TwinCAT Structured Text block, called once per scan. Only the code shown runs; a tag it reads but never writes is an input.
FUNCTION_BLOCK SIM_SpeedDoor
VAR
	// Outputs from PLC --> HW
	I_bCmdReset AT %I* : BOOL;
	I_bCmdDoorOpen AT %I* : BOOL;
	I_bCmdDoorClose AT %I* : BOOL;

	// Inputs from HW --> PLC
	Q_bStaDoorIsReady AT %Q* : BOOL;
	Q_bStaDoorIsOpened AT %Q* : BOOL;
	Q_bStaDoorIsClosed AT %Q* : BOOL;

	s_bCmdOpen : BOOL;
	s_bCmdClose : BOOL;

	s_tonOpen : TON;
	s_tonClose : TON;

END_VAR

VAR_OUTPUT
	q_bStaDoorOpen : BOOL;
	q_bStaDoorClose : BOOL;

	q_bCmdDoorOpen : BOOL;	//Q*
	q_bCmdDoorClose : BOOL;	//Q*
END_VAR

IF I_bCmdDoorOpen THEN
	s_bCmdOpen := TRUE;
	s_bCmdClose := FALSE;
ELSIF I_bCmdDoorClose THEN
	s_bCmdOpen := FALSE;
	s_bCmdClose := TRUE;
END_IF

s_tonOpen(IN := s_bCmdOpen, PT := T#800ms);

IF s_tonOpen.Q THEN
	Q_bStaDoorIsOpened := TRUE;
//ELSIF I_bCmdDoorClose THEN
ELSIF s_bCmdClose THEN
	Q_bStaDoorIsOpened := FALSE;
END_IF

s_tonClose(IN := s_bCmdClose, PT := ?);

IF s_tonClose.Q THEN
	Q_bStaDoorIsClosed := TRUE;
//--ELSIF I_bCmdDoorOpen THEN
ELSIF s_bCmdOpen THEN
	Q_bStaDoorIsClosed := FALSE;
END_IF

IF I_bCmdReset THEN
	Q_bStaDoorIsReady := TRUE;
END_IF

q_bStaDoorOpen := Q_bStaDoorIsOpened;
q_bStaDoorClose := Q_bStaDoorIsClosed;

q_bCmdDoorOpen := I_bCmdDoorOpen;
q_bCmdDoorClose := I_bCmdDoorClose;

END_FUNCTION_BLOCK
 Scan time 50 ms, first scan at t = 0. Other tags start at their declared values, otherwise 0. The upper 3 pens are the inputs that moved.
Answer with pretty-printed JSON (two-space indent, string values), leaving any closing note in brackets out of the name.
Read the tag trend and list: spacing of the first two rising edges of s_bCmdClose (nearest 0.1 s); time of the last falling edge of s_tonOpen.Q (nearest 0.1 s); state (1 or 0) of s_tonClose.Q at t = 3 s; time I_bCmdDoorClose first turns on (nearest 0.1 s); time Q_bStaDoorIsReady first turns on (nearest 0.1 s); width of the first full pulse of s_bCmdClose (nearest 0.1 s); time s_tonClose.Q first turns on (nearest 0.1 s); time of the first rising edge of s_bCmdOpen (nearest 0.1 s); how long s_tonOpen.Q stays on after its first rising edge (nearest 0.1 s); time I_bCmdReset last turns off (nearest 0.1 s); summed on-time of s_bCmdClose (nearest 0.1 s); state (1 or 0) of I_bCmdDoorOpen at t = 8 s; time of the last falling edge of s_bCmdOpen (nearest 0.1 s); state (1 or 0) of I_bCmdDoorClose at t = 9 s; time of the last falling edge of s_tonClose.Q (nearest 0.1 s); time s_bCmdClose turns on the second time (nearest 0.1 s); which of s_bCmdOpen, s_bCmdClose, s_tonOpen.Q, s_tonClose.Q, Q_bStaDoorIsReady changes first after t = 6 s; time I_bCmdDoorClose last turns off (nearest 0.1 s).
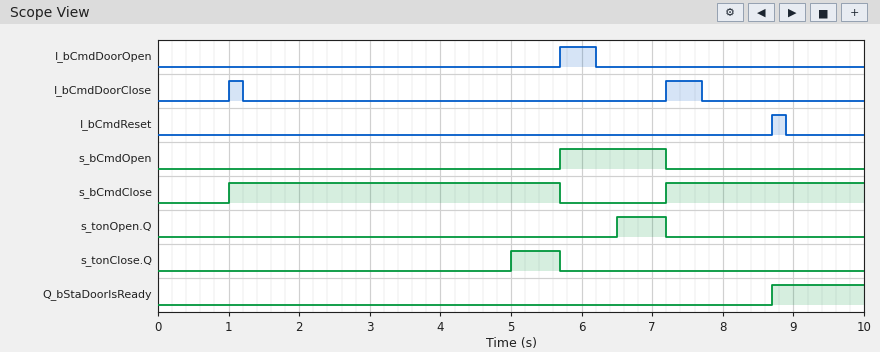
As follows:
{
  "spacing of the first two rising edges of s_bCmdClose": "6.2 s",
  "time of the last falling edge of s_tonOpen.Q": "7.2 s",
  "state (1 or 0) of s_tonClose.Q at t = 3 s": "0",
  "time I_bCmdDoorClose first turns on": "1.0 s",
  "time Q_bStaDoorIsReady first turns on": "8.7 s",
  "width of the first full pulse of s_bCmdClose": "4.7 s",
  "time s_tonClose.Q first turns on": "5.0 s",
  "time of the first rising edge of s_bCmdOpen": "5.7 s",
  "how long s_tonOpen.Q stays on after its first rising edge": "0.7 s",
  "time I_bCmdReset last turns off": "8.9 s",
  "summed on-time of s_bCmdClose": "7.5 s",
  "state (1 or 0) of I_bCmdDoorOpen at t = 8 s": "0",
  "time of the last falling edge of s_bCmdOpen": "7.2 s",
  "state (1 or 0) of I_bCmdDoorClose at t = 9 s": "0",
  "time of the last falling edge of s_tonClose.Q": "5.7 s",
  "time s_bCmdClose turns on the second time": "7.2 s",
  "which of s_bCmdOpen, s_bCmdClose, s_tonOpen.Q, s_tonClose.Q, Q_bStaDoorIsReady changes first after t = 6 s": "s_tonOpen.Q",
  "time I_bCmdDoorClose last turns off": "7.7 s"
}
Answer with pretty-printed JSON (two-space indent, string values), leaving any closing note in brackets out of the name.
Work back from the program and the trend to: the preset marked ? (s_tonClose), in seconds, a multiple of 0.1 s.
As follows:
{
  "the preset marked ? (s_tonClose), in seconds, a multiple of 0.1 s": "4.0 s"
}
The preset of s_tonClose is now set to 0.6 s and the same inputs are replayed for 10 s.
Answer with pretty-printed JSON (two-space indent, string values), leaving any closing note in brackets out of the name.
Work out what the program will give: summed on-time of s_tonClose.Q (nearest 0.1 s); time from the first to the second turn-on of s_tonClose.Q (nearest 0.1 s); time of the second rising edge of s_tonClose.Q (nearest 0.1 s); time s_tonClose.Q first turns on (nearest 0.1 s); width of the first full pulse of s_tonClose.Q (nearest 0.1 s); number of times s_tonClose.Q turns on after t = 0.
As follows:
{
  "summed on-time of s_tonClose.Q": "6.3 s",
  "time from the first to the second turn-on of s_tonClose.Q": "6.2 s",
  "time of the second rising edge of s_tonClose.Q": "7.8 s",
  "time s_tonClose.Q first turns on": "1.6 s",
  "width of the first full pulse of s_tonClose.Q": "4.1 s",
  "number of times s_tonClose.Q turns on after t = 0": "2"
}
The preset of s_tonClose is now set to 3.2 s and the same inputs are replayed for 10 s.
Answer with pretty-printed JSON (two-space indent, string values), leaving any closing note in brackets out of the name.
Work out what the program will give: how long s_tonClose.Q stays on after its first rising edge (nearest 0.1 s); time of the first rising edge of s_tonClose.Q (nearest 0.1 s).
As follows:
{
  "how long s_tonClose.Q stays on after its first rising edge": "1.5 s",
  "time of the first rising edge of s_tonClose.Q": "4.2 s"
}
